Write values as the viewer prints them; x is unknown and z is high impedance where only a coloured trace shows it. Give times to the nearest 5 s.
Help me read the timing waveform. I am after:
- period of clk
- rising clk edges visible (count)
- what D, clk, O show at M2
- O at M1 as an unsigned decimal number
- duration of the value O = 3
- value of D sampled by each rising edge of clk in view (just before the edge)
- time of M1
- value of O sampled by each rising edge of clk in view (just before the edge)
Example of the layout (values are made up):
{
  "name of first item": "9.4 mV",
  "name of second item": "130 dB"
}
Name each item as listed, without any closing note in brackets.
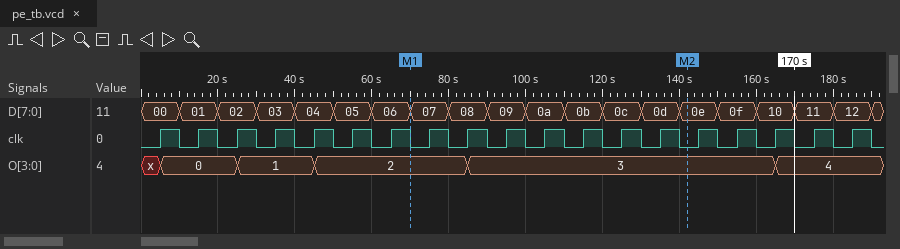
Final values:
{
  "period of clk": "10 s",
  "rising clk edges visible": "19",
  "what D, clk, O show at M2": "D=0e, clk=0, O=3",
  "O at M1 as an unsigned decimal number": "2",
  "duration of the value O = 3": "80 s",
  "value of D sampled by each rising edge of clk in view": "00, 01, 02, 03, 04, 05, 06, 07, 08, 09, 0a, 0b, 0c, 0d, 0e, 0f, 10, 11, 12",
  "time of M1": "70 s",
  "value of O sampled by each rising edge of clk in view": "x, 0, 0, 1, 1, 2, 2, 2, 2, 3, 3, 3, 3, 3, 3, 3, 3, 4, 4"
}
